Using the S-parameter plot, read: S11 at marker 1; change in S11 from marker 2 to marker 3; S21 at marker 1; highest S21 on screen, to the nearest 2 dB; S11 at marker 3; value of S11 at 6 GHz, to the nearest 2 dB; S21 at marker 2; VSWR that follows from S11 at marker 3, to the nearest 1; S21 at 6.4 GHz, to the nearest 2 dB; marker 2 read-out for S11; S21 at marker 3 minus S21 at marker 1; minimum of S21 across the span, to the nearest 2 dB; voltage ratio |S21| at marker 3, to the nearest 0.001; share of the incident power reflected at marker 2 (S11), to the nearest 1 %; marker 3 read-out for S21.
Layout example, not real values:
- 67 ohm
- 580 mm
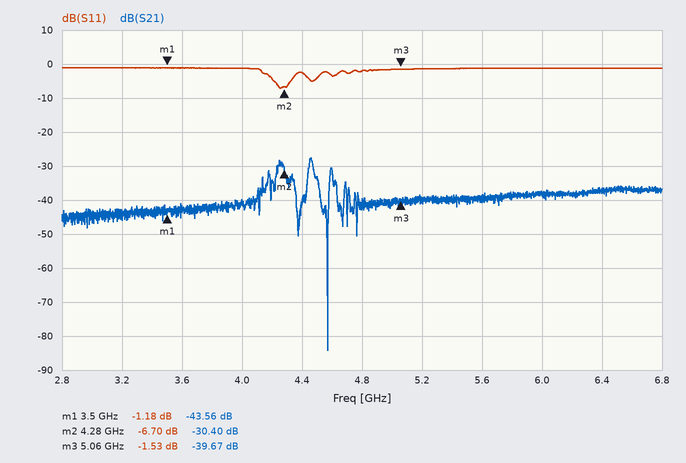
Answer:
- -1.18 dB
- 5.17 dB
- -43.56 dB
- -28 dB
- -1.53 dB
- -2 dB
- -30.40 dB
- 11
- -38 dB
- -6.70 dB
- 3.89 dB
- -84 dB
- 0.010
- 21 %
- -39.67 dB
